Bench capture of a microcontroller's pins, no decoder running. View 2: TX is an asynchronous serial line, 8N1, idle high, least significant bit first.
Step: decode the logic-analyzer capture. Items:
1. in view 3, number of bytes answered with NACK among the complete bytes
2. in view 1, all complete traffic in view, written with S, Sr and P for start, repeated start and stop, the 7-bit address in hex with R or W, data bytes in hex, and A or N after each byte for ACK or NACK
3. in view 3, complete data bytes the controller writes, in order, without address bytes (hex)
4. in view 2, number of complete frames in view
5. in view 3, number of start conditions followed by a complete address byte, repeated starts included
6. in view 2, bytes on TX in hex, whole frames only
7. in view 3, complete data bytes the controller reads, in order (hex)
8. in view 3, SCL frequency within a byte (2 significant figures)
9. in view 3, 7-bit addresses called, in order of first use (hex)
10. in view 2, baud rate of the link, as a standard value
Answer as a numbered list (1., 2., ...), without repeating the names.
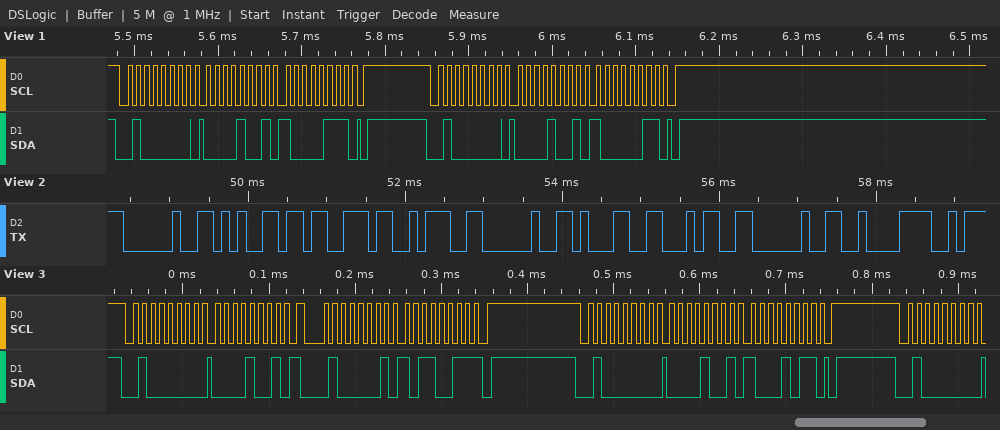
1. 1
2. S 20W A 09 A 87 A P S 20W A 09 A 83 A P
3. 09 09 8B
4. 9
5. 4
6. 20 65 73 3A 20 31 34 20 C2
7. B3
8. 100 kHz
9. 0x20
10. 9600 baud
